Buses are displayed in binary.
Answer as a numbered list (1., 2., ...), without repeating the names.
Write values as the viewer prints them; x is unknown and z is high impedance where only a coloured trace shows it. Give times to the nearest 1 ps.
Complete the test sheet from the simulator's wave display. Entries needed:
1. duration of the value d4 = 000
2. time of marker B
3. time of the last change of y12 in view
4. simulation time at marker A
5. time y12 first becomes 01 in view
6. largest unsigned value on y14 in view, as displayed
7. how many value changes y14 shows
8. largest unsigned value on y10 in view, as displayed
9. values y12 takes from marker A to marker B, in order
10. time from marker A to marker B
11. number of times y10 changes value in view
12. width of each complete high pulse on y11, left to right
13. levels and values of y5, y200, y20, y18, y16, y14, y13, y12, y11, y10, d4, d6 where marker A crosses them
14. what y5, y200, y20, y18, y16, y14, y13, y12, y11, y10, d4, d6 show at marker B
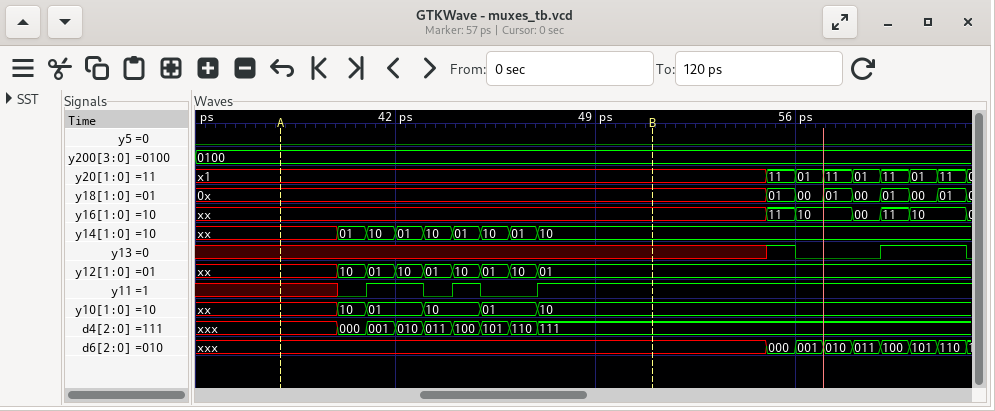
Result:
1. 1 ps
2. 51 ps
3. 47 ps
4. 38 ps
5. 41 ps
6. 10
7. 8
8. 10
9. xx, 10, 01, 10, 01, 10, 01, 10, 01
10. 13 ps
11. 5
12. 2 ps, 1 ps
13. y5=0, y200=0100, y20=x1, y18=0x, y16=xx, y14=xx, y13=x, y12=xx, y11=x, y10=xx, d4=xxx, d6=xxx
14. y5=0, y200=0100, y20=x1, y18=0x, y16=xx, y14=10, y13=x, y12=01, y11=1, y10=10, d4=111, d6=xxx
